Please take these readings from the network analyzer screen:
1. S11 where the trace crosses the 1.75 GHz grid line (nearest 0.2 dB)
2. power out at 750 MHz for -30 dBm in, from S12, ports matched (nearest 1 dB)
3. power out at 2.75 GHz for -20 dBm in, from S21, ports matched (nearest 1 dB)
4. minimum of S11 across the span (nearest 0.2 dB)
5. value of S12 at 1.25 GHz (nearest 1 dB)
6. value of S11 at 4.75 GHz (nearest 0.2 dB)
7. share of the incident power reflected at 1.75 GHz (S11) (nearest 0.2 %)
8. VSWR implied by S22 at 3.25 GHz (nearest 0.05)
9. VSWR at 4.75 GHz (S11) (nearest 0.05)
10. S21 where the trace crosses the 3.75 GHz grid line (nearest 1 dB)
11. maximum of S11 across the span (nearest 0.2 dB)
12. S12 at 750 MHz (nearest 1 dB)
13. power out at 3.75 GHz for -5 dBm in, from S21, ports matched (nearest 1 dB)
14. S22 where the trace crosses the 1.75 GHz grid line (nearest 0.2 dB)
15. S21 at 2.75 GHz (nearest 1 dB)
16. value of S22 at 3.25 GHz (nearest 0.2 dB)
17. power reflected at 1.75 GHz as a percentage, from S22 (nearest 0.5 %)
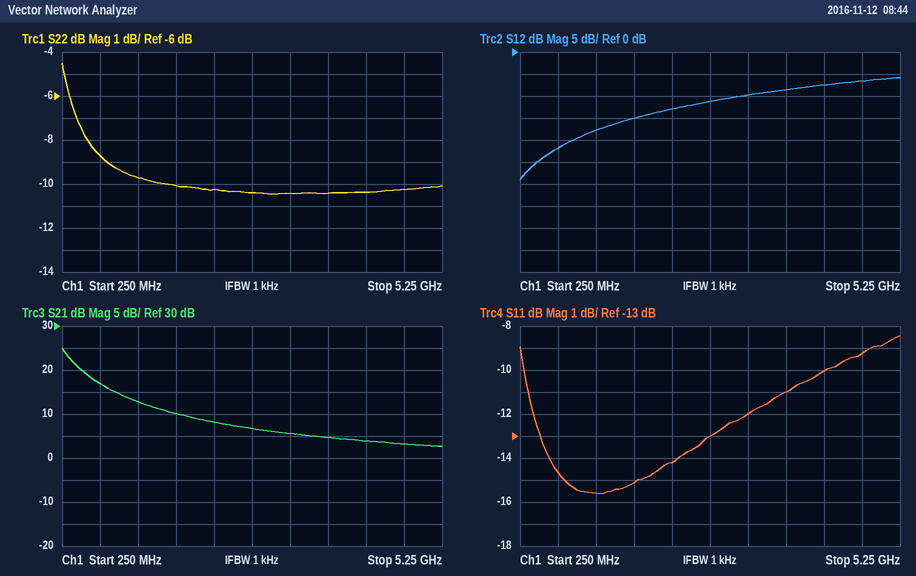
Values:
-15.2 dB
-52 dBm
-13 dBm
-15.6 dB
-18 dB
-9.2 dB
3.0 %
1.85
2.05
5 dB
-8.4 dB
-22 dB
0 dBm
-10.0 dB
7 dB
-10.4 dB
10.0 %
